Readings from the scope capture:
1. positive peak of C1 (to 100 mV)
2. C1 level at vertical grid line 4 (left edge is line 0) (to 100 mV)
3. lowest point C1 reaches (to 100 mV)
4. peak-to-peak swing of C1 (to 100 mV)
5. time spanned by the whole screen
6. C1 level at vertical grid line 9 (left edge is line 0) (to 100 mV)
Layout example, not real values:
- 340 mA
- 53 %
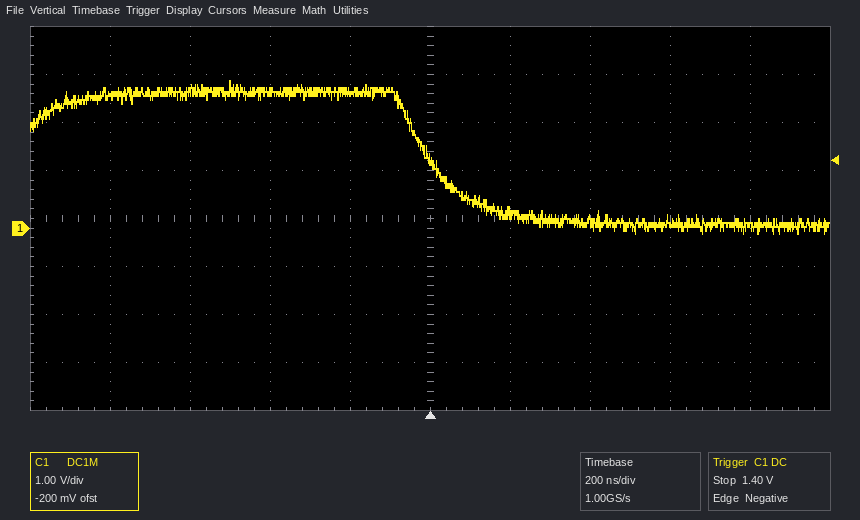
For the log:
- 3.1 V
- 2.8 V
- -100 mV
- 3.2 V
- 2 µs
- 0.0 V
